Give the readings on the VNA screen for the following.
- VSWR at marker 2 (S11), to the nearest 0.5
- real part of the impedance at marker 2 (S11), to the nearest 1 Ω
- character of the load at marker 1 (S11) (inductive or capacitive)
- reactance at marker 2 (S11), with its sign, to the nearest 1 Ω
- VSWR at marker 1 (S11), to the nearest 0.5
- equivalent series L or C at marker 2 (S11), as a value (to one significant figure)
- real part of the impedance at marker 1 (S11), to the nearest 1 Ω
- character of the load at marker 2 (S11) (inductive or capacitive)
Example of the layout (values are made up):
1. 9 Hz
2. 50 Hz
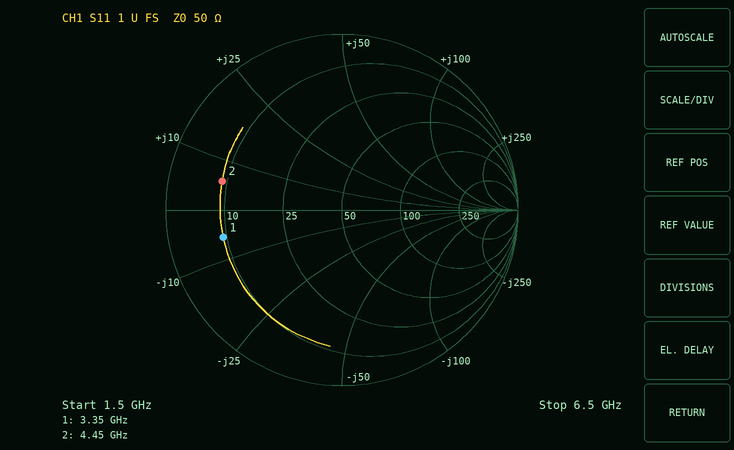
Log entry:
1. 5.5
2. 9 Ω
3. capacitive
4. +6 Ω
5. 5.5
6. 200 pH
7. 9 Ω
8. inductive
